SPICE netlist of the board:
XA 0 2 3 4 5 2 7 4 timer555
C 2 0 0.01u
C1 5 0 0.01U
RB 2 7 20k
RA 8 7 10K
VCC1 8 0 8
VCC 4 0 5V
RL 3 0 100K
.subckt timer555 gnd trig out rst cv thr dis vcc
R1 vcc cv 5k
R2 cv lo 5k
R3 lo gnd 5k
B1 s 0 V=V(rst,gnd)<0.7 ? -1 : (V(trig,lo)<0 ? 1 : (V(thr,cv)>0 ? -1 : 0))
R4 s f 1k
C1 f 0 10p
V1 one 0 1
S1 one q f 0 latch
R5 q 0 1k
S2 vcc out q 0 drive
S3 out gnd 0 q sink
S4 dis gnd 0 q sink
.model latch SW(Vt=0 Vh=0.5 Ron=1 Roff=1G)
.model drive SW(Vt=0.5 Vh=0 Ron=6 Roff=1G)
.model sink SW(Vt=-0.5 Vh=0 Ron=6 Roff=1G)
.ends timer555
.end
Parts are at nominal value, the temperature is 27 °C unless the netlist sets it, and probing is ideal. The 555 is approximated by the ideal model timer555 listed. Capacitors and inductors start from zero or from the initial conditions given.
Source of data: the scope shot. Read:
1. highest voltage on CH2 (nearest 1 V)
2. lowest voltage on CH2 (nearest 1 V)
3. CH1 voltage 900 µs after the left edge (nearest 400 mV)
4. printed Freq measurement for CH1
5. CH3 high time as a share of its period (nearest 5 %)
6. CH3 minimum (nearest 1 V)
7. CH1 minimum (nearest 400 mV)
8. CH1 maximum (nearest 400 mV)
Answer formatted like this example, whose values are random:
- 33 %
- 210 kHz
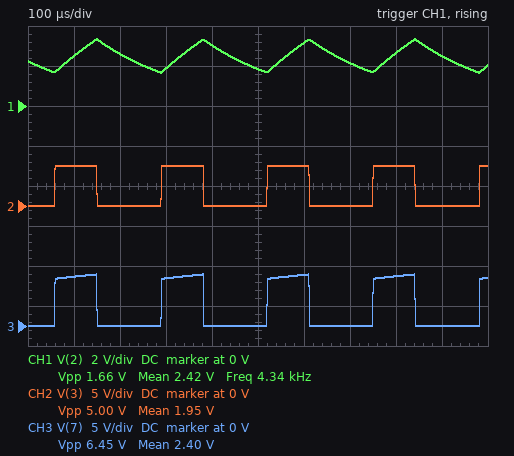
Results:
- 5 V
- 0 V
- 2.4 V
- 4.34 kHz
- 40 %
- 0 V
- 1.6 V
- 3.2 V
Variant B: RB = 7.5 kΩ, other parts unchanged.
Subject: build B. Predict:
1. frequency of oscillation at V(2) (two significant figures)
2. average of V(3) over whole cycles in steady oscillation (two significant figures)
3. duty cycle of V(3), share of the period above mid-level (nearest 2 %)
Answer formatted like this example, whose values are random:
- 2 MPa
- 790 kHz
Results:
- 9.5 kHz
- 2.5 V
- 50 %
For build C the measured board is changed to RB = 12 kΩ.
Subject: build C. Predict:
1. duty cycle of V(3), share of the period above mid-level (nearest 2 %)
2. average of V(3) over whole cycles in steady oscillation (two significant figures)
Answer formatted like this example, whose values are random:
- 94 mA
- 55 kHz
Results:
- 44 %
- 2.2 V
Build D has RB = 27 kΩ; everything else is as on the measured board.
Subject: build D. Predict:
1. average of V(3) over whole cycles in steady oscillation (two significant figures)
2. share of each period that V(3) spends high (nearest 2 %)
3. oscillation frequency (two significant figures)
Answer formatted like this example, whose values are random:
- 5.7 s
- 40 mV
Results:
- 1.9 V
- 38 %
- 3.3 kHz
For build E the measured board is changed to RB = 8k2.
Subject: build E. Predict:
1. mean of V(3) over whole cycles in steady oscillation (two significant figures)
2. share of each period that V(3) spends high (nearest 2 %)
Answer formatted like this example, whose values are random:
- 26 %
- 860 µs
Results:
- 2.5 V
- 50 %
